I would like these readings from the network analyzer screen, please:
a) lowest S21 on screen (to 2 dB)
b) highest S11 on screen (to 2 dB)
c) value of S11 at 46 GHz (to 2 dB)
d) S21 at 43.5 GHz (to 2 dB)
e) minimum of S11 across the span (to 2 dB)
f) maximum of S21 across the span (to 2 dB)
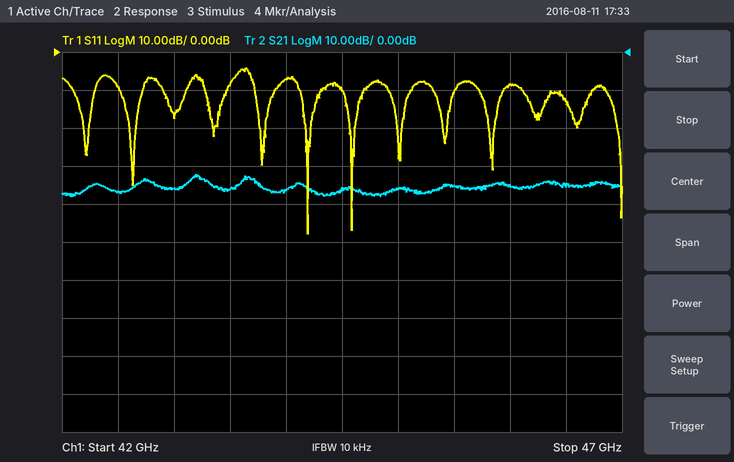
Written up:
-38 dB
-4 dB
-8 dB
-36 dB
-48 dB
-32 dB
